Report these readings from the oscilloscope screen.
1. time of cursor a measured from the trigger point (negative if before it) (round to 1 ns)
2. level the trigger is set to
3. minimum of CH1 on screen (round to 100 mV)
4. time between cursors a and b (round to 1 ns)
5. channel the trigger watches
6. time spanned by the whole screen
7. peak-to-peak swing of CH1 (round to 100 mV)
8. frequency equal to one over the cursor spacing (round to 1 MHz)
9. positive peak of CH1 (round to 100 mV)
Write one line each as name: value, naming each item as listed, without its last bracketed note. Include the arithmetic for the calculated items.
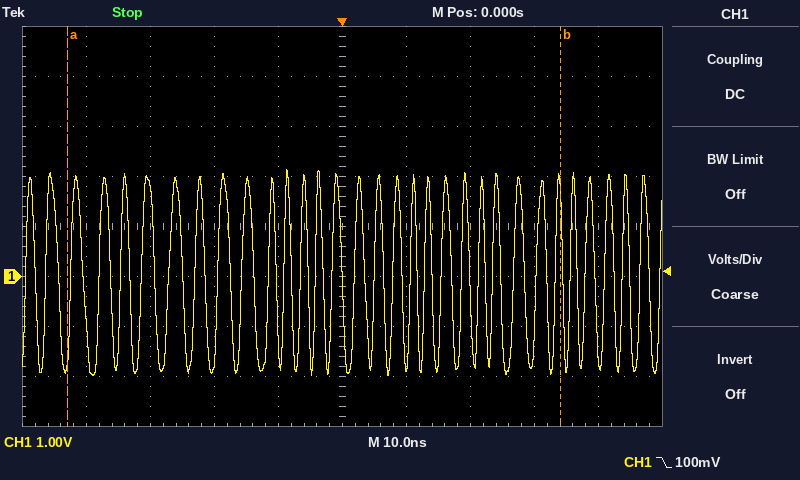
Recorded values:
time of cursor a measured from the trigger point (negative if before it): -43 ns
level the trigger is set to: 100 mV
minimum of CH1 on screen: -2.0 V
time between cursors a and b: 77 ns
channel the trigger watches: CH1
time spanned by the whole screen: 100 ns
peak-to-peak swing of CH1: 2.1 V − (-2.0 V) = 4.1 V
frequency equal to one over the cursor spacing: 1 / 77 ns ≈ 13 MHz
positive peak of CH1: 2.1 V
